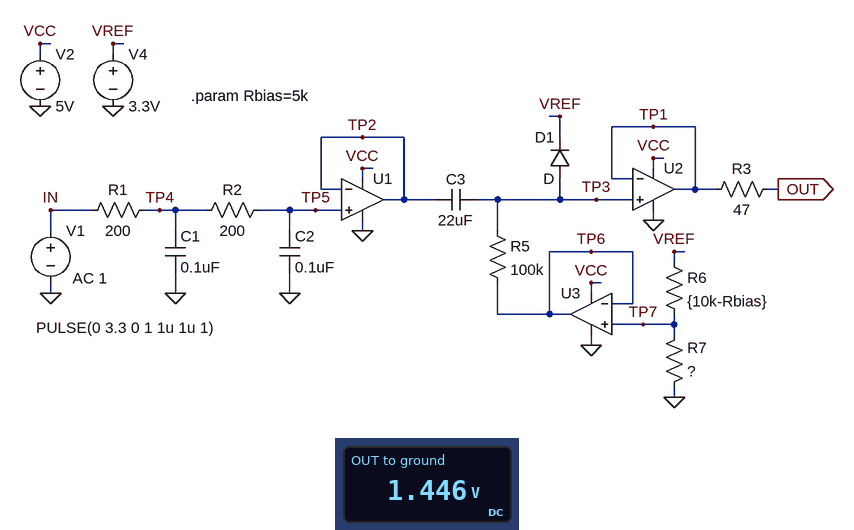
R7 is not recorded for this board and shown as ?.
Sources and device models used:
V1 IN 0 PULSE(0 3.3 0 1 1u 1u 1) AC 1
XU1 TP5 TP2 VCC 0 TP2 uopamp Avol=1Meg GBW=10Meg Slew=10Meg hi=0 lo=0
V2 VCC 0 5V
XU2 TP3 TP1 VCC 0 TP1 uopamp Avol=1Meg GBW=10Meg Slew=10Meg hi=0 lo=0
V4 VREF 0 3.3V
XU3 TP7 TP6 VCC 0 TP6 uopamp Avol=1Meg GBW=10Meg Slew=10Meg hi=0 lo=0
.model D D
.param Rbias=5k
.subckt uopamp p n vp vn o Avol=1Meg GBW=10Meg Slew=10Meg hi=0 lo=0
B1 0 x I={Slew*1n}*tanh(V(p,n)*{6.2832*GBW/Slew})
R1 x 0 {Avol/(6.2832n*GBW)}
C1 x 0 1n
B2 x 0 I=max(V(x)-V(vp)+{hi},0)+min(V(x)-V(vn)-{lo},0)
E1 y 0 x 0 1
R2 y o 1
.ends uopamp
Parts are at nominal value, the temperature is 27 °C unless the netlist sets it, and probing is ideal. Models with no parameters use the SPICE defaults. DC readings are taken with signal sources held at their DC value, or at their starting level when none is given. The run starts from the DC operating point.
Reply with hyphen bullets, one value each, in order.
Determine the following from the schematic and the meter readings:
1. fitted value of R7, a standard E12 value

- 3.9 kΩ
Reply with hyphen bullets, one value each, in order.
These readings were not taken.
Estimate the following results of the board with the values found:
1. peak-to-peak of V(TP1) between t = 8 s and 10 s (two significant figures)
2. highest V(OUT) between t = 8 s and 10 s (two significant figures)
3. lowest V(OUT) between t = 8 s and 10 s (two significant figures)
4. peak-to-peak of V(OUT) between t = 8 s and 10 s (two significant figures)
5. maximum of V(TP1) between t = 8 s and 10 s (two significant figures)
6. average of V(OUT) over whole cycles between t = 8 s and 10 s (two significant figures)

- 3.0 V
- 3.0 V
- -9.5 mV
- 3.0 V
- 3.0 V
- 1.5 V
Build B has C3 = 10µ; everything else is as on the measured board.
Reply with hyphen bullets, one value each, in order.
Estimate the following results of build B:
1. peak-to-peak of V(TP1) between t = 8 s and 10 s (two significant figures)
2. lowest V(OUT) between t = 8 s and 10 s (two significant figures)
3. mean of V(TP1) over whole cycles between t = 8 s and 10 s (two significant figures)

- 2.8 V
- -9.9 mV
- 1.5 V
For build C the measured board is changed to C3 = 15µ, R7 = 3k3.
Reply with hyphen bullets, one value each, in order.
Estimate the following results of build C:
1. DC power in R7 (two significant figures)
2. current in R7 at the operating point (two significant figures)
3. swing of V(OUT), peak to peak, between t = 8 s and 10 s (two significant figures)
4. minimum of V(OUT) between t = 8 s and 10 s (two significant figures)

- 520 µW
- 400 µA
- 2.8 V
- -10 mV
